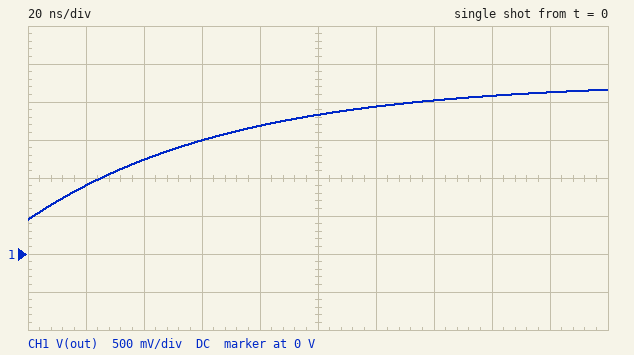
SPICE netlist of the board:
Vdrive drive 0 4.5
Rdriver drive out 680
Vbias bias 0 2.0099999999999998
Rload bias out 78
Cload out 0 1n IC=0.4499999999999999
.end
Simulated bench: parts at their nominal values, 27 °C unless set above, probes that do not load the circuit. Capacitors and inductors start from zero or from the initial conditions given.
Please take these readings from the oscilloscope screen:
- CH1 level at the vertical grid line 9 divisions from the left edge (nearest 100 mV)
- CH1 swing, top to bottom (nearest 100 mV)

2.1 V
1.7 V
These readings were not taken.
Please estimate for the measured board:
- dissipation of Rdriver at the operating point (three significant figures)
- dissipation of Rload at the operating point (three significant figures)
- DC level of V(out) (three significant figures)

7.34 mW
842 µW
2.27 V
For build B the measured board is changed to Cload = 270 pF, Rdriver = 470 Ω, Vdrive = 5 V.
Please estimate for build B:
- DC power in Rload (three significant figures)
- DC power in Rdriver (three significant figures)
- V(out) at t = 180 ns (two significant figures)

2.32 mW
14.0 mW
2.4 V
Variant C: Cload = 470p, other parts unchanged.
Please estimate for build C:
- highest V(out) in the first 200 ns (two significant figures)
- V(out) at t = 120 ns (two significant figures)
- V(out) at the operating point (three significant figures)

2.3 V
2.2 V
2.27 V
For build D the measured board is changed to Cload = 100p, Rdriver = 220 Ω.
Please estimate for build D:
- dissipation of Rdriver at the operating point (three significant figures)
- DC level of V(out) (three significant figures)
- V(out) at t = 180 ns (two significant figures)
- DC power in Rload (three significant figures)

15.4 mW
2.66 V
2.7 V
5.45 mW
